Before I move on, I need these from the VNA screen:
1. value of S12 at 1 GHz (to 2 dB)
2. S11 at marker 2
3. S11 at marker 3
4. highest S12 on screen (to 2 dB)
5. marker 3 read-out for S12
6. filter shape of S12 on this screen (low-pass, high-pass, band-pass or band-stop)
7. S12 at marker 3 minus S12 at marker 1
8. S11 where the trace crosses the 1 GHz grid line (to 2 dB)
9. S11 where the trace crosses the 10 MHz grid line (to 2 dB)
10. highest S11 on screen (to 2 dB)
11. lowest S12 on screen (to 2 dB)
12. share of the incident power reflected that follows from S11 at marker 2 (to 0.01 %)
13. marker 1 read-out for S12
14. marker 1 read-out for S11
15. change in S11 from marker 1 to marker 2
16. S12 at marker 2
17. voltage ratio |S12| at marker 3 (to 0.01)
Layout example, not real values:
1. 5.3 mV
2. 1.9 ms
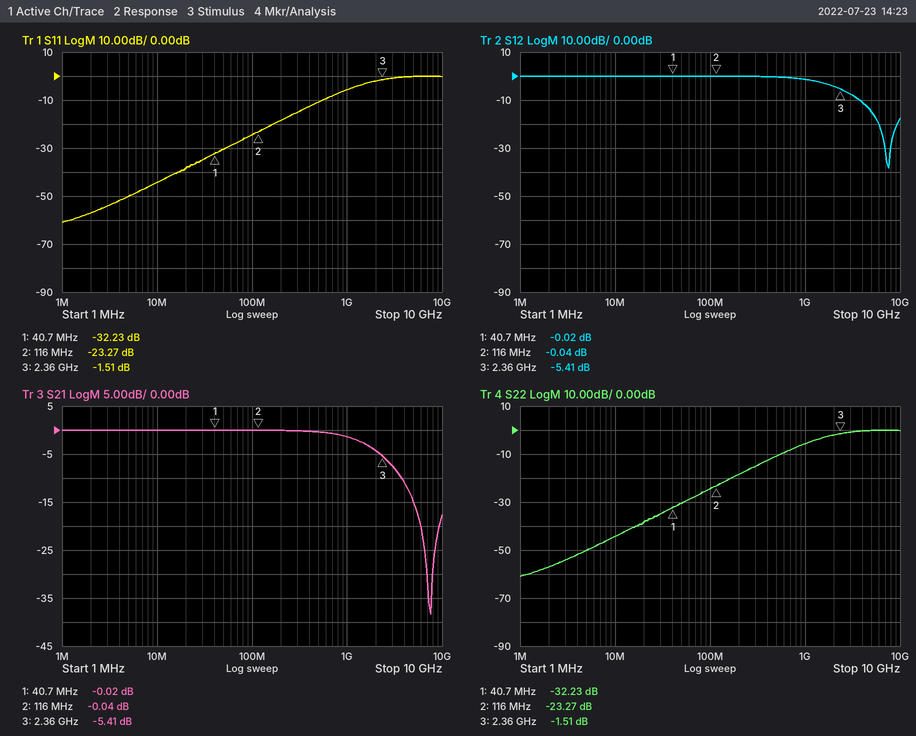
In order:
1. -2 dB
2. -23.27 dB
3. -1.51 dB
4. 0 dB
5. -5.41 dB
6. low-pass
7. -5.39 dB
8. -6 dB
9. -44 dB
10. 0 dB
11. -38 dB
12. 0.47 %
13. -0.02 dB
14. -32.23 dB
15. 8.96 dB
16. -0.04 dB
17. 0.54
